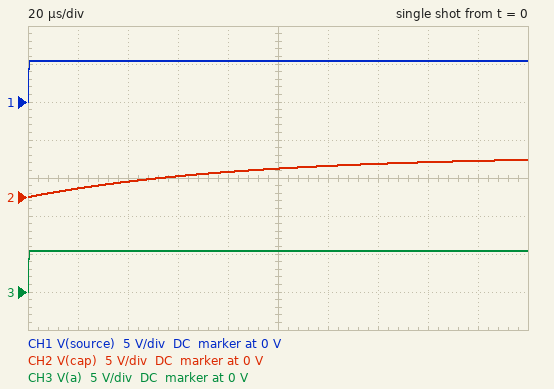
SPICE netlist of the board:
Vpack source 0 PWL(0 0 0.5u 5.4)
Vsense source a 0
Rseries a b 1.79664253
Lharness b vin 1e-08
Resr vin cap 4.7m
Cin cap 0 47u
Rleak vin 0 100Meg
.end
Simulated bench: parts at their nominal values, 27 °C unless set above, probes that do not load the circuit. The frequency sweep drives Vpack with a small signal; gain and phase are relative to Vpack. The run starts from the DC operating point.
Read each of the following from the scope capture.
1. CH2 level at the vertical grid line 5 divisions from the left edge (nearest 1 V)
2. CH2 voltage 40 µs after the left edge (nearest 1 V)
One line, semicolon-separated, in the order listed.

4 V; 2 V
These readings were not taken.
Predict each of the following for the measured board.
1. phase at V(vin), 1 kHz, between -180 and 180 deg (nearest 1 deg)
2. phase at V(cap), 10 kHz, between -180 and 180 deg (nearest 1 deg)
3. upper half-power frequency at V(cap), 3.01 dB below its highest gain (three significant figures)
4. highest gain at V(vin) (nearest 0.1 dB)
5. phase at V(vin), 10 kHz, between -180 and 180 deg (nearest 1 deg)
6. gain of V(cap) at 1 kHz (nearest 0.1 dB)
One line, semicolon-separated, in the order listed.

-28 deg; -79 deg; 1.88 kHz; 0 dB; -79 deg; -1.1 dB
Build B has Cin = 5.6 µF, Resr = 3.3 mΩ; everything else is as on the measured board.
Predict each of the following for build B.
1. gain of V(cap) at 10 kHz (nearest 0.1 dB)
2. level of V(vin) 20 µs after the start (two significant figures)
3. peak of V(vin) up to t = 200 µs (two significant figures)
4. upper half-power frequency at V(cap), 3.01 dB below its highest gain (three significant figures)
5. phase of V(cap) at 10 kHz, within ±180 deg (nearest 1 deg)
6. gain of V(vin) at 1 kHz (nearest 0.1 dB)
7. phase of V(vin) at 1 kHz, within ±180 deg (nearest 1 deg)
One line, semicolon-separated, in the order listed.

-1.5 dB; 4.6 V; 5.4 V; 15.8 kHz; -32 deg; 0 dB; -4 deg
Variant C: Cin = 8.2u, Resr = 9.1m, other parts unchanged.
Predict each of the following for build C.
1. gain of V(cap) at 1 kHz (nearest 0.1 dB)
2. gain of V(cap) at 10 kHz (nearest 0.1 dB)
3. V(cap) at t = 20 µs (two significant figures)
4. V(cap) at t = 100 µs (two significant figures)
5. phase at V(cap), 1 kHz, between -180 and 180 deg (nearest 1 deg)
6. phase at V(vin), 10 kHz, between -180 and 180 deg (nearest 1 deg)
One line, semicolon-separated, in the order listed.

0 dB; -2.7 dB; 4.0 V; 5.4 V; -5 deg; -43 deg
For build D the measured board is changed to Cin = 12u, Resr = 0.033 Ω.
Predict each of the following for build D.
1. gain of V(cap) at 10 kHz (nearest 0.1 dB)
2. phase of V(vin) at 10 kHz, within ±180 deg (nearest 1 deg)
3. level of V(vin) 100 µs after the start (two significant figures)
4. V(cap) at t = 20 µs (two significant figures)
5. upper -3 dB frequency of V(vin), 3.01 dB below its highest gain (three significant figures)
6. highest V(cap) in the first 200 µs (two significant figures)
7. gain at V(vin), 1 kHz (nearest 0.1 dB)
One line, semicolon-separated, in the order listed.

-4.6 dB; -53 deg; 5.3 V; 3.2 V; 7.25 kHz; 5.4 V; -0.1 dB
